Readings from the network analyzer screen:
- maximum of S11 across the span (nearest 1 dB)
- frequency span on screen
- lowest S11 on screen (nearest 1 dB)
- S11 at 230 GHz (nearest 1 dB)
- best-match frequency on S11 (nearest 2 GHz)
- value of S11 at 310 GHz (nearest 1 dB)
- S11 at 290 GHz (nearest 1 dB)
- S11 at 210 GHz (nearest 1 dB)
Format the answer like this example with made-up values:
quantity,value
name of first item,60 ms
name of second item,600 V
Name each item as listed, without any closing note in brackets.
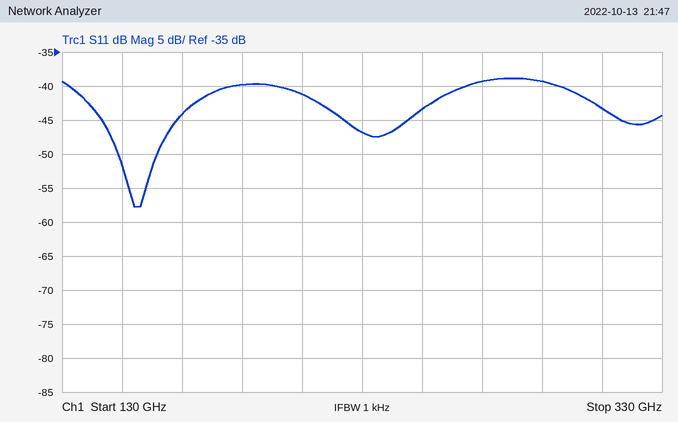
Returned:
quantity,value
maximum of S11 across the span,-39 dB
frequency span on screen,200 GHz
lowest S11 on screen,-58 dB
S11 at 230 GHz,-47 dB
best-match frequency on S11,154 GHz
value of S11 at 310 GHz,-43 dB
S11 at 290 GHz,-39 dB
S11 at 210 GHz,-41 dB
